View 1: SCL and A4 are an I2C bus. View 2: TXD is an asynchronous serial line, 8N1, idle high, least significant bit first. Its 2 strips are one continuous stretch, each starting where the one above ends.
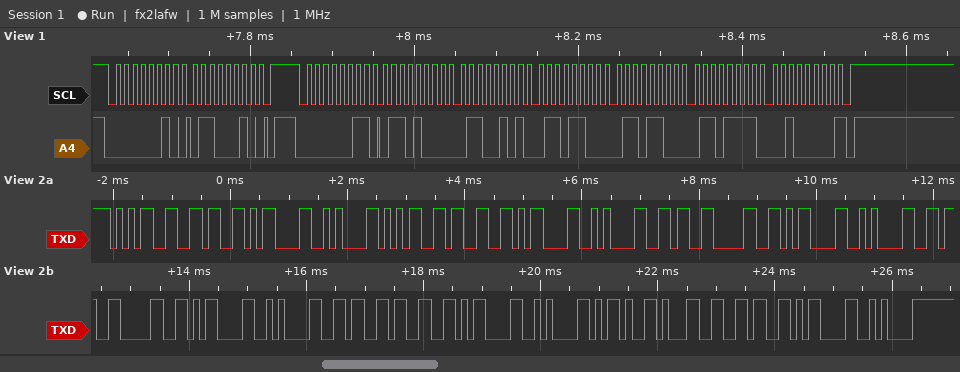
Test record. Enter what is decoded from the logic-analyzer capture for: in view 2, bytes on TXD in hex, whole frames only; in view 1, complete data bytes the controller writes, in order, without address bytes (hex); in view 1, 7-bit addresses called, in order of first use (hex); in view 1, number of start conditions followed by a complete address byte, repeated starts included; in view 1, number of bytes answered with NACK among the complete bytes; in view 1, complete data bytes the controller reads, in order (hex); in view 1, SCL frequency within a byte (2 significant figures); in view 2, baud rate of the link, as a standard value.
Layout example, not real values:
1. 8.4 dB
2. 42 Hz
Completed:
1. 35 36 0D 0A 35 33 0D 0A 36 30 0D 0A 36 30 0D 0A 36 33 0D 0A 2D 31 36 0D 0A
2. 62
3. 0x01
4. 2
5. 1
6. 68 65 6C 6C 6F 20
7. 100 kHz
8. 9600 baud
